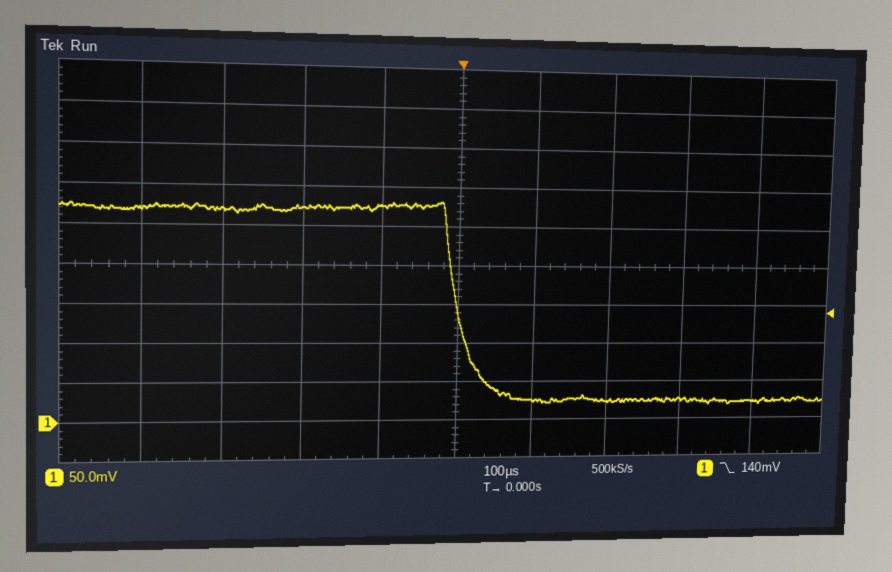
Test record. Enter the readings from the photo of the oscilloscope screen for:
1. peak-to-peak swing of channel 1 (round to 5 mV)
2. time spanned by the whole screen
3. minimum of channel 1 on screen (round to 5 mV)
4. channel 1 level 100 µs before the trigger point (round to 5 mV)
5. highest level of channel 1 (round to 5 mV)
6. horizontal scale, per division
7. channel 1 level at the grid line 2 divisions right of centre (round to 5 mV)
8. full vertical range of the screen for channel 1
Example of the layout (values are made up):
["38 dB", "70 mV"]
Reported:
["260 mV", "1 ms", "20 mV", "275 mV", "280 mV", "100 µs", "25 mV", "500 mV"]
